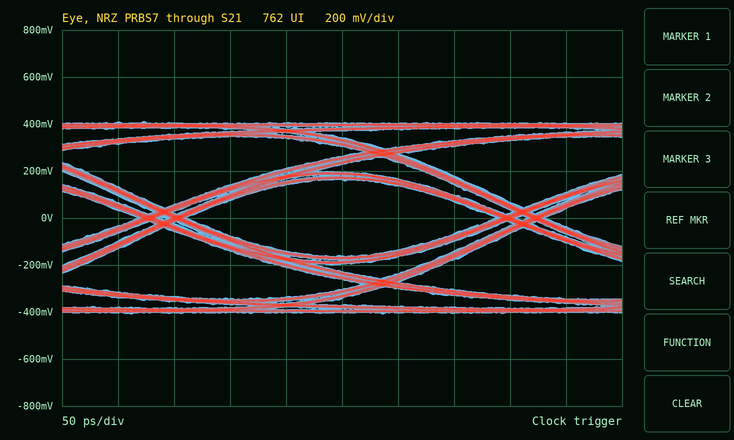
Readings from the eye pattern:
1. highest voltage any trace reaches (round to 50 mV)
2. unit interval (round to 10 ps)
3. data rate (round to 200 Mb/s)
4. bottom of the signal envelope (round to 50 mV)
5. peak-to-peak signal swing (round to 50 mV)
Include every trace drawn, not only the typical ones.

400 mV
320 ps
3.2 Gb/s
-400 mV
800 mV
